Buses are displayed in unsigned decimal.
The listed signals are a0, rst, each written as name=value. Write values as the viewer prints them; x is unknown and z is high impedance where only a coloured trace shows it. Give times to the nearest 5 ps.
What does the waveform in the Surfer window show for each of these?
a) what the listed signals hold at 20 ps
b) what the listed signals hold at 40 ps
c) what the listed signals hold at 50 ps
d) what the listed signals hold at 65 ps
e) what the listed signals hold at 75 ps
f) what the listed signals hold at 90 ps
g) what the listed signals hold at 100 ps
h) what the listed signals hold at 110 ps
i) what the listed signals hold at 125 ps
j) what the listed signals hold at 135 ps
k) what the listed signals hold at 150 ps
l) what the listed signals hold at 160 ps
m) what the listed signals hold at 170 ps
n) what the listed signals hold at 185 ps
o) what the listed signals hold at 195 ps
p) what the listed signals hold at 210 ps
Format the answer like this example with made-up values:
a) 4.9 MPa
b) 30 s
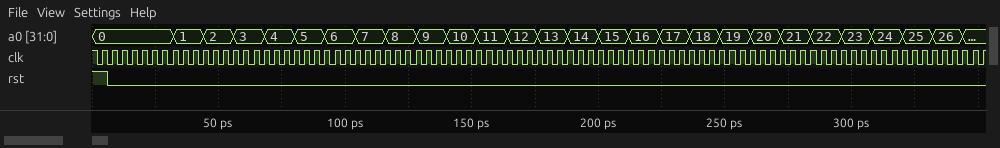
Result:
a) a0=0, rst=0
b) a0=1, rst=0
c) a0=2, rst=0
d) a0=3, rst=0
e) a0=4, rst=0
f) a0=5, rst=0
g) a0=6, rst=0
h) a0=7, rst=0
i) a0=8, rst=0
j) a0=9, rst=0
k) a0=10, rst=0
l) a0=11, rst=0
m) a0=12, rst=0
n) a0=13, rst=0
o) a0=14, rst=0
p) a0=15, rst=0
